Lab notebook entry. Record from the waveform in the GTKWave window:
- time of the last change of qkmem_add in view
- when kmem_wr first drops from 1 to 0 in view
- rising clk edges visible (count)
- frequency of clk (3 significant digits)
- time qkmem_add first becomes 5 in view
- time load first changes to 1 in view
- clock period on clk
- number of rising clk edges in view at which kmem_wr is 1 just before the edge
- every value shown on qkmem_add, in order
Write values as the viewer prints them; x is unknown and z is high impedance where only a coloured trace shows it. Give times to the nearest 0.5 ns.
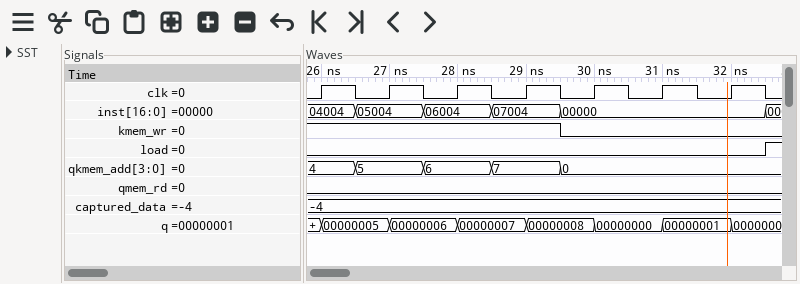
29.5 ns
29.5 ns
7
1.00 GHz
26.5 ns
32.5 ns
1 ns
4
4, 5, 6, 7, 0
